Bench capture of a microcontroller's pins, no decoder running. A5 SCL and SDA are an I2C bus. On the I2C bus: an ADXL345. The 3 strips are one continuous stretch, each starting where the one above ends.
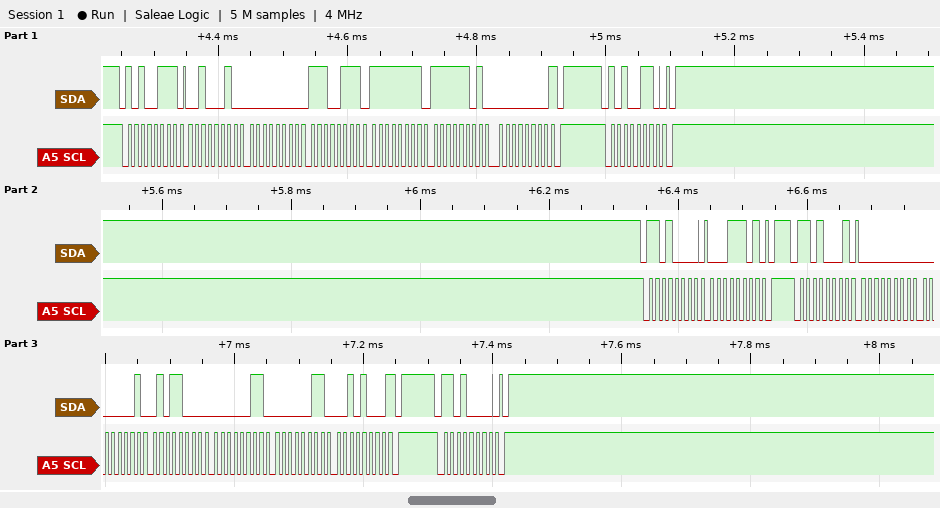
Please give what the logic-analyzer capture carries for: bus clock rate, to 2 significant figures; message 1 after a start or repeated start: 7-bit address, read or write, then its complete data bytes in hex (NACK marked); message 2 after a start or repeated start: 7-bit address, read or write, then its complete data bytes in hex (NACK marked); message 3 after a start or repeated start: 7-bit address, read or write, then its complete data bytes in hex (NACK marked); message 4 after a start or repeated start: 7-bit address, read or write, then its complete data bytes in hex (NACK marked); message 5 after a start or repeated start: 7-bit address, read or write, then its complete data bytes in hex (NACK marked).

100 kHz
0x53 read: 22 00 E7 FF FD 00 NACK
0x53 write
0x68 write: 1D
0x68 read: 00 01 58 03 03 28 NACK
0x68 write
